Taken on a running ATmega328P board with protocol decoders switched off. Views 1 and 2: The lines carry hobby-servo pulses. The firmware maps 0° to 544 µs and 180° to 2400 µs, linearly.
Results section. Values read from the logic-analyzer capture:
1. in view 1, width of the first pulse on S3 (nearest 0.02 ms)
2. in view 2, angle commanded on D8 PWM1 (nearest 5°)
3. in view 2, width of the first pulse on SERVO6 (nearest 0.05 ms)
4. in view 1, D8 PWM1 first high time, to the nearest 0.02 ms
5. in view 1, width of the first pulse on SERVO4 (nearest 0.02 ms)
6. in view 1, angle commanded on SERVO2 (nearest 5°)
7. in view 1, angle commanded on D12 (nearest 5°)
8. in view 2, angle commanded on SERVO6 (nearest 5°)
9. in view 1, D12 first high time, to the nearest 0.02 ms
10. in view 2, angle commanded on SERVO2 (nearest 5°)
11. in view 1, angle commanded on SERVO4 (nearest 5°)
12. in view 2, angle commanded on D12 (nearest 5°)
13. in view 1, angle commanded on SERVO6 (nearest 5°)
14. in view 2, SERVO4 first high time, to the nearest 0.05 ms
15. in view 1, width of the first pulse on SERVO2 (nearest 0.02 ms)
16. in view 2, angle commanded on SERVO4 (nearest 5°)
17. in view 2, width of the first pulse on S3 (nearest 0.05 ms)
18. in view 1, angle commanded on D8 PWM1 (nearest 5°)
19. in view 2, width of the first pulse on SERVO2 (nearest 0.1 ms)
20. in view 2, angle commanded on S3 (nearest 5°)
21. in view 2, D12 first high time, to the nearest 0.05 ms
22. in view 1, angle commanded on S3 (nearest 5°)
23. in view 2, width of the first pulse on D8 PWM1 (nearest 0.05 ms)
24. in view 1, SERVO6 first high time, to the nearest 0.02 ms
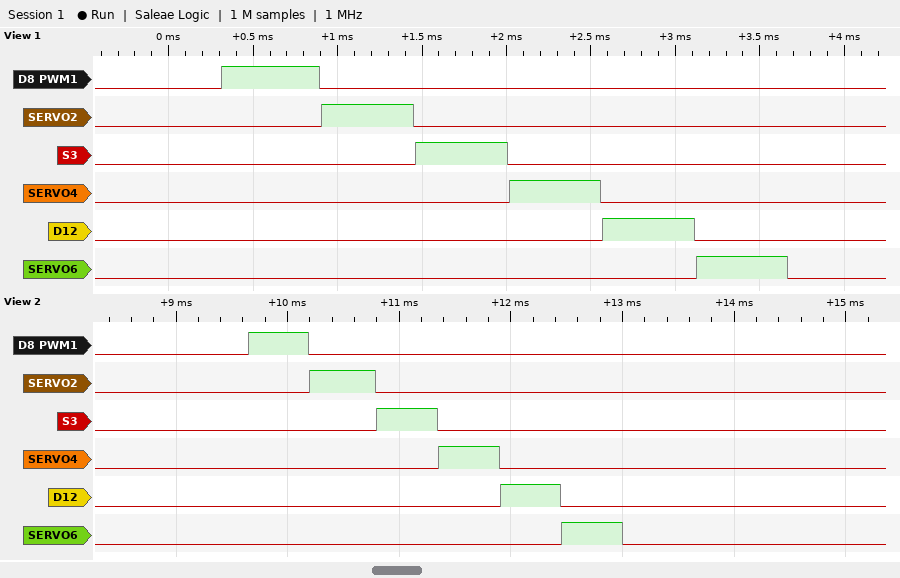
0.54 ms
0°
0.55 ms
0.58 ms
0.54 ms
0°
0°
0°
0.54 ms
5°
0°
0°
0°
0.55 ms
0.54 ms
0°
0.55 ms
5°
0.6 ms
0°
0.55 ms
0°
0.55 ms
0.54 ms
